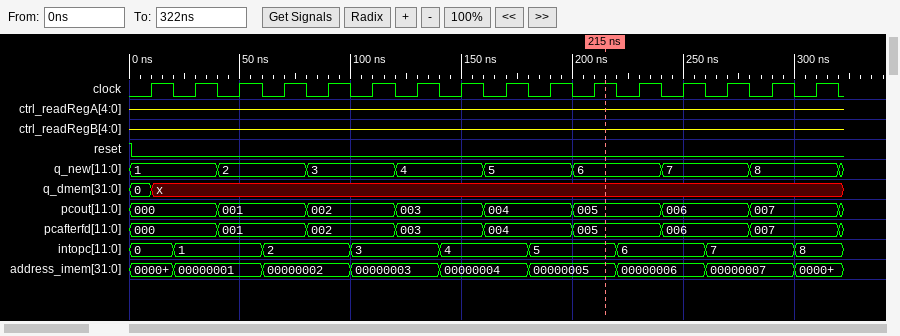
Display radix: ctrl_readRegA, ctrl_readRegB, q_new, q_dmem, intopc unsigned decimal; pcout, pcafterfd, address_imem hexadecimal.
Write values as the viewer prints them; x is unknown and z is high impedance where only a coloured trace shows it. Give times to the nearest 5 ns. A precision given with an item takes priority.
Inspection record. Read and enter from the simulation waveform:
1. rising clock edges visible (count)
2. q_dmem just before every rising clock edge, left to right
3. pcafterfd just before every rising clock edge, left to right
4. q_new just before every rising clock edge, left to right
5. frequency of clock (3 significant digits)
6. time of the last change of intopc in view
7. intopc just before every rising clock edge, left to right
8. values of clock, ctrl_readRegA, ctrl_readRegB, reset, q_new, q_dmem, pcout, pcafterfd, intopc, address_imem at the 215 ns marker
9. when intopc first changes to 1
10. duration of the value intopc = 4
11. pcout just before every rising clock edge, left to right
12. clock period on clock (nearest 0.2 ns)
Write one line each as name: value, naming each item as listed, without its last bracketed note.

rising clock edges visible: 16
q_dmem just before every rising clock edge, left to right: 0, x, x, x, x, x, x, x, x, x, x, x, x, x, x, x
pcafterfd just before every rising clock edge, left to right: 000, 000, 001, 001, 002, 002, 003, 003, 004, 004, 005, 005, 006, 006, 007, 007
q_new just before every rising clock edge, left to right: 1, 1, 2, 2, 3, 3, 4, 4, 5, 5, 6, 6, 7, 7, 8, 8
frequency of clock: 50.0 MHz
time of the last change of intopc in view: 300 ns
intopc just before every rising clock edge, left to right: 0, 1, 1, 2, 2, 3, 3, 4, 4, 5, 5, 6, 6, 7, 7, 8
values of clock, ctrl_readRegA, ctrl_readRegB, reset, q_new, q_dmem, pcout, pcafterfd, intopc, address_imem at the 215 ns marker: clock=1, ctrl_readRegA=z, ctrl_readRegB=z, reset=0, q_new=6, q_dmem=x, pcout=005, pcafterfd=005, intopc=5, address_imem=00000005
when intopc first changes to 1: 20 ns
duration of the value intopc = 4: 40 ns
pcout just before every rising clock edge, left to right: 000, 000, 001, 001, 002, 002, 003, 003, 004, 004, 005, 005, 006, 006, 007, 007
clock period on clock: 20 ns
